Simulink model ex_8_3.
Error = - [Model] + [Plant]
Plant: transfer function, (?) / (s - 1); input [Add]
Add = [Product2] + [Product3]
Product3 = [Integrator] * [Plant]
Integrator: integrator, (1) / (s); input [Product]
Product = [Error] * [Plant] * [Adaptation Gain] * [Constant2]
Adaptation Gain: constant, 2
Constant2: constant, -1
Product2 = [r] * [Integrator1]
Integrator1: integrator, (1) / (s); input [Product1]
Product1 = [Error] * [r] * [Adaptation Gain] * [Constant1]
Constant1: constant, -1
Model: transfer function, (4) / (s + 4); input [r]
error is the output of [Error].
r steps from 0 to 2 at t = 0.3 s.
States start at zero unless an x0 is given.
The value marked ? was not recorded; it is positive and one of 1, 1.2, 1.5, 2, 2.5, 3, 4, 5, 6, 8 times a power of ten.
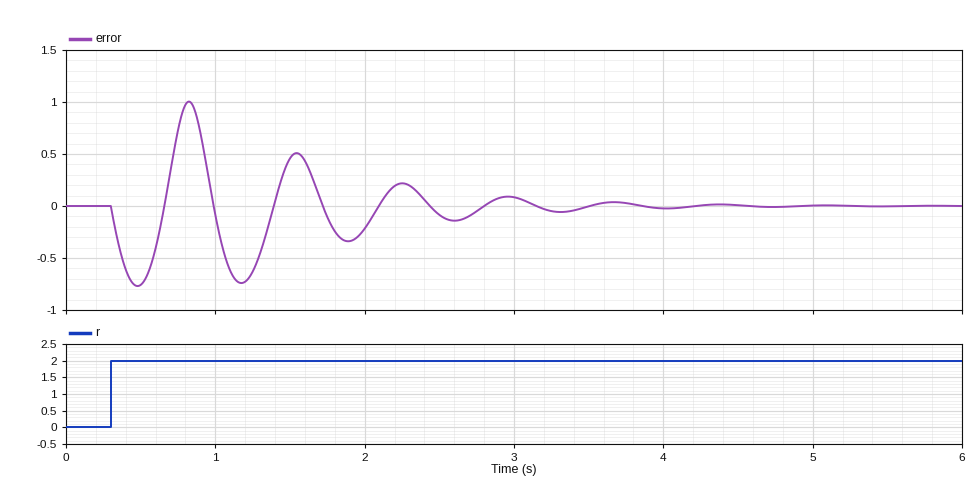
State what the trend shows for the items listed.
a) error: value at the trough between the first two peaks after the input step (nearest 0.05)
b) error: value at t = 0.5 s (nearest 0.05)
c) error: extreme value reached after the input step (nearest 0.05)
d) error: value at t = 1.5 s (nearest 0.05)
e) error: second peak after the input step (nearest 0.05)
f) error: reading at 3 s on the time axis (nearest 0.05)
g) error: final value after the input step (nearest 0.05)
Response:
-0.75
-0.75
1.00
0.45
0.50
0.10
0.00
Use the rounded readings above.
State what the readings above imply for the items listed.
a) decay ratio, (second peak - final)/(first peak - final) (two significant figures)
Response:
0.50
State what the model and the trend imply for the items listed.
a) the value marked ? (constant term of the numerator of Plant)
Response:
5
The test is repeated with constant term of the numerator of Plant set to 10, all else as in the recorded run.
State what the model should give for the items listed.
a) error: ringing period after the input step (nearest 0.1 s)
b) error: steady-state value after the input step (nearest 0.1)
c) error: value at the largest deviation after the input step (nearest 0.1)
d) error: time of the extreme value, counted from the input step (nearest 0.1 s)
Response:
0.5 s
0.0
0.8
0.4 s
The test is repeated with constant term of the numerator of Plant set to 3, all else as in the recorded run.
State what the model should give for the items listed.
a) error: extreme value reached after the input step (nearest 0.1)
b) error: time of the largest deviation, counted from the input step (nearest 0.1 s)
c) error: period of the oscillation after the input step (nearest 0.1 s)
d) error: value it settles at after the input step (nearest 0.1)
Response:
1.2
0.6 s
0.9 s
0.0
